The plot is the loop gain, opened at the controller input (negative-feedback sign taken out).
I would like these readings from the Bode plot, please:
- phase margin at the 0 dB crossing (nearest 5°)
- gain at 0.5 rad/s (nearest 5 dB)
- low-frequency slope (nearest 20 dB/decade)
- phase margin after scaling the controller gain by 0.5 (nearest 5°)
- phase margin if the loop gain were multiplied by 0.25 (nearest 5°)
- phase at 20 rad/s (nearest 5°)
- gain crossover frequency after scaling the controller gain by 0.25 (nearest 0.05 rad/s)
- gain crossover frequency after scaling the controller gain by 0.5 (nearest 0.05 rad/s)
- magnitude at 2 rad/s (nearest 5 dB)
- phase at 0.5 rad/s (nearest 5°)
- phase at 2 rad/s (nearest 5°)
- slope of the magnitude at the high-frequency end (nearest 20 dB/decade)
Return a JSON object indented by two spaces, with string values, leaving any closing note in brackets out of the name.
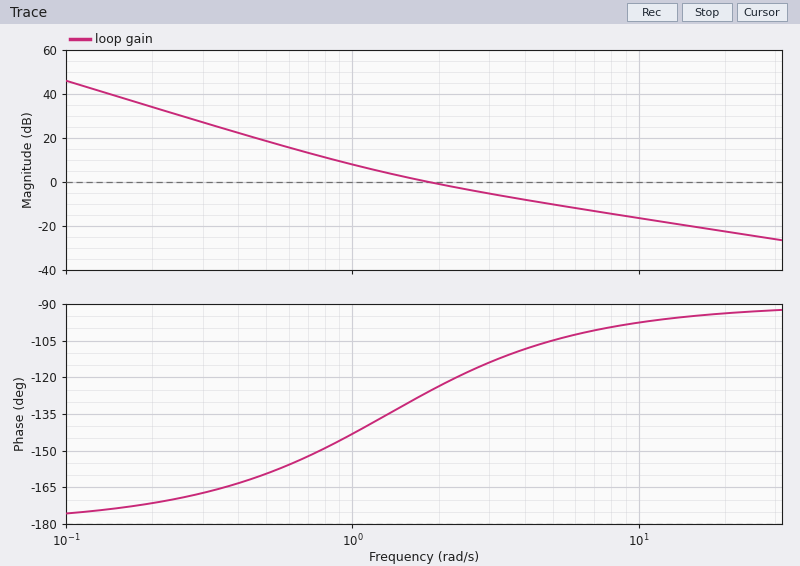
{
  "phase margin at the 0 dB crossing": "55°",
  "gain at 0.5 rad/s": "20 dB",
  "low-frequency slope": "-40 dB/decade",
  "phase margin after scaling the controller gain by 0.5": "40°",
  "phase margin if the loop gain were multiplied by 0.25": "30°",
  "phase at 20 rad/s": "-95°",
  "gain crossover frequency after scaling the controller gain by 0.25": "0.75 rad/s",
  "gain crossover frequency after scaling the controller gain by 0.5": "1.15 rad/s",
  "magnitude at 2 rad/s": "0 dB",
  "phase at 0.5 rad/s": "-160°",
  "phase at 2 rad/s": "-125°",
  "slope of the magnitude at the high-frequency end": "-20 dB/decade"
}
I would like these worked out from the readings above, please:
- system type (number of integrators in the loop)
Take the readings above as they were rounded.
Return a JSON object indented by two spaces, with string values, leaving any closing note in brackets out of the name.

{
  "system type": "2"
}
